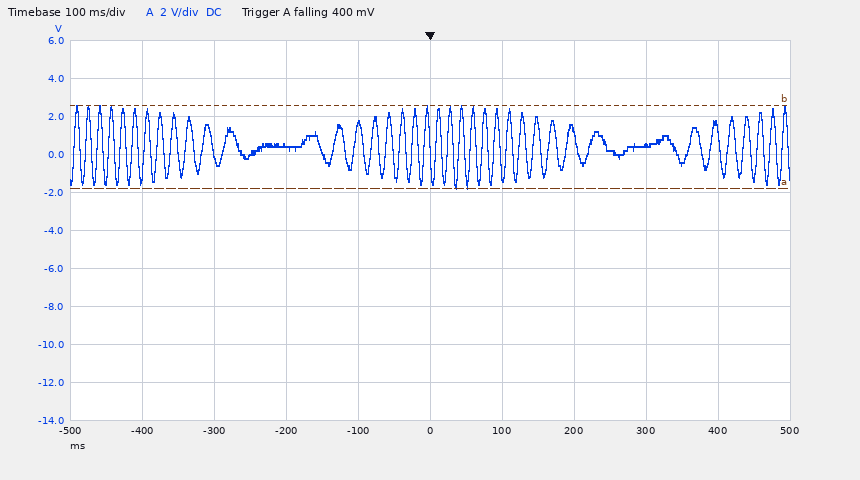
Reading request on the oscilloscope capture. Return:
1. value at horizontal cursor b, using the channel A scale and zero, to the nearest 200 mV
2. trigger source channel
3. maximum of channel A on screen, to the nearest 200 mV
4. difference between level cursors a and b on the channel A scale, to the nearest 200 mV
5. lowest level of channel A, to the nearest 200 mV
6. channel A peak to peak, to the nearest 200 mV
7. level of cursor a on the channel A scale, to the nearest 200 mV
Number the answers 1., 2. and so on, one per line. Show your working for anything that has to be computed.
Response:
1. 2.6 V
2. channel A
3. 2.6 V
4. 4.4 V
5. -1.8 V
6. 2.6 V − (-1.8 V) = 4.4 V
7. -1.8 V
